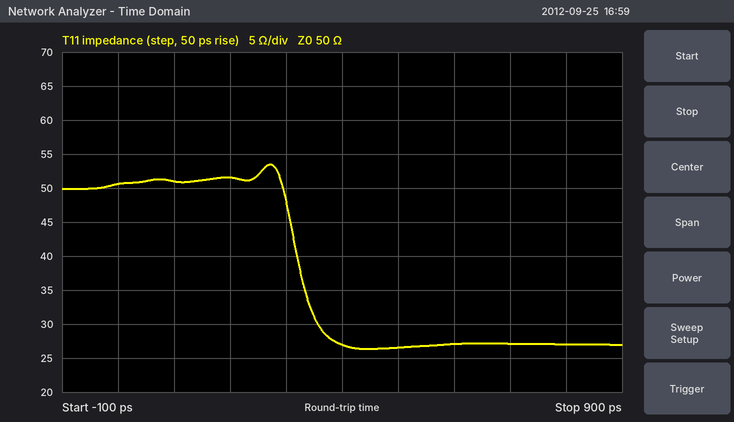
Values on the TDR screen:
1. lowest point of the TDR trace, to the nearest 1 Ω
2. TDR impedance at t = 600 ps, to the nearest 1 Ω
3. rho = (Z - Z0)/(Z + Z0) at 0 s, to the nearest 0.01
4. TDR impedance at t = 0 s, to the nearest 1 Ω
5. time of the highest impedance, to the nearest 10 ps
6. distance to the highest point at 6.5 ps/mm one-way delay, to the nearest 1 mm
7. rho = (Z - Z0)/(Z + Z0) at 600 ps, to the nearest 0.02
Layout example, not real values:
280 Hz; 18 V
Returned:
26 Ω; 27 Ω; +0.01; 51 Ω; 270 ps; 21 mm; -0.30
